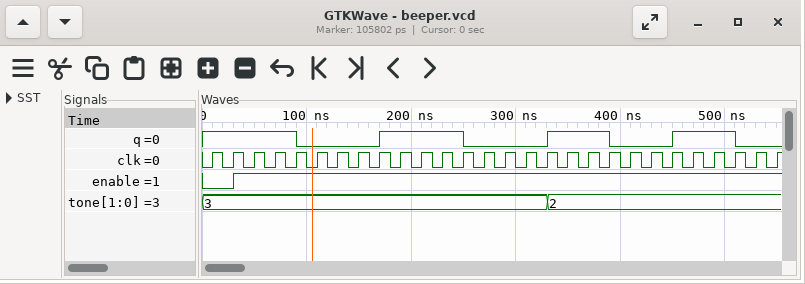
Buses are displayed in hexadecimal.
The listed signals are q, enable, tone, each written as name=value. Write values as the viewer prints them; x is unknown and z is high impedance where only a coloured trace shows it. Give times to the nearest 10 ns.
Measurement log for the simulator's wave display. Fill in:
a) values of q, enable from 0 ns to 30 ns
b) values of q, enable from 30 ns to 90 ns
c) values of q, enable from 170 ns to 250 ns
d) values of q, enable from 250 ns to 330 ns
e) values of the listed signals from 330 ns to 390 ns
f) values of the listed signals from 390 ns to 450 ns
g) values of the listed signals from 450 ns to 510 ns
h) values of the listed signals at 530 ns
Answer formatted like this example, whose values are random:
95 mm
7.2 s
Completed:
q=1, enable=0
q=1, enable=1
q=1, enable=1
q=0, enable=1
q=1, enable=1, tone=2
q=0, enable=1, tone=2
q=1, enable=1, tone=2
q=0, enable=1, tone=2
